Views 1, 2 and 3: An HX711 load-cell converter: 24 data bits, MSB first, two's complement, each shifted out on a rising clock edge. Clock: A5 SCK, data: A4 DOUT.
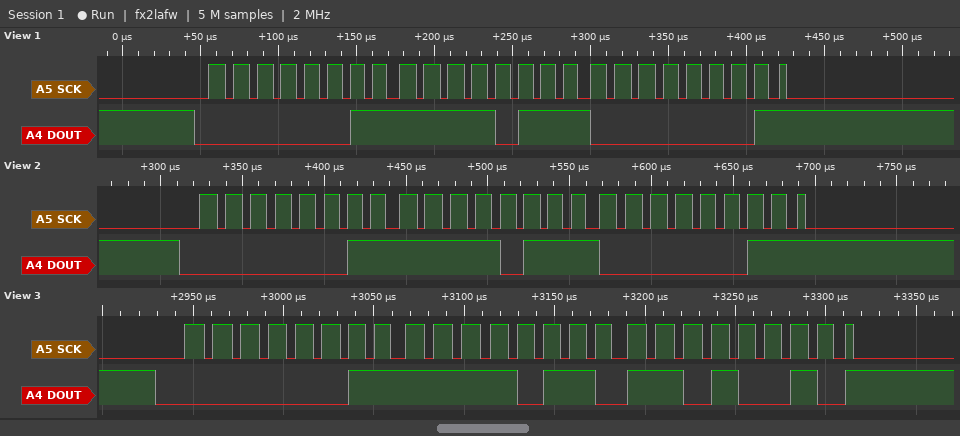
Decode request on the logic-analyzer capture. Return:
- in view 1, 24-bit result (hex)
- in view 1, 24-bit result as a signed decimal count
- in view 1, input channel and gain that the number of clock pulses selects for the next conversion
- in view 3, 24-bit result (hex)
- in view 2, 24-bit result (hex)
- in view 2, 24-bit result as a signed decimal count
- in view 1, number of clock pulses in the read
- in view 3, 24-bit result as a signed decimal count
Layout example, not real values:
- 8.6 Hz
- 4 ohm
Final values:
- 0x03F701
- 259841
- channel A, gain 128
- 0x03F6D2
- 0x03F703
- 259843
- 25
- 259794
